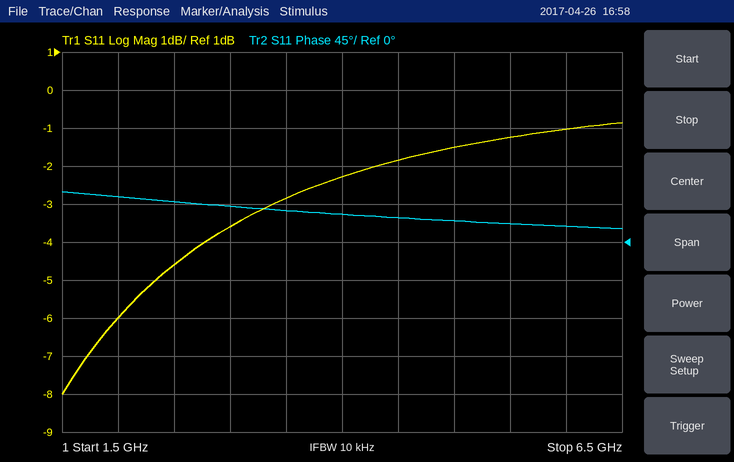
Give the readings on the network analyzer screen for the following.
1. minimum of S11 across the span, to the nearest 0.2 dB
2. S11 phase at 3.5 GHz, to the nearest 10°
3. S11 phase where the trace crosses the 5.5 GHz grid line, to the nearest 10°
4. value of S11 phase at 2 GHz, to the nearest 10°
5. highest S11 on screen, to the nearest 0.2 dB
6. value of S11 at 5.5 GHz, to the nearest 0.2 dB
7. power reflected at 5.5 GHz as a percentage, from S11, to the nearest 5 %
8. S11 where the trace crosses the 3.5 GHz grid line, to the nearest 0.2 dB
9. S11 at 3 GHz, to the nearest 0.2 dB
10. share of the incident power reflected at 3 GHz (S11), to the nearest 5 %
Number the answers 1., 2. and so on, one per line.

1. -8.0 dB
2. 40°
3. 20°
4. 50°
5. -0.8 dB
6. -1.2 dB
7. 75 %
8. -2.8 dB
9. -3.6 dB
10. 45 %
